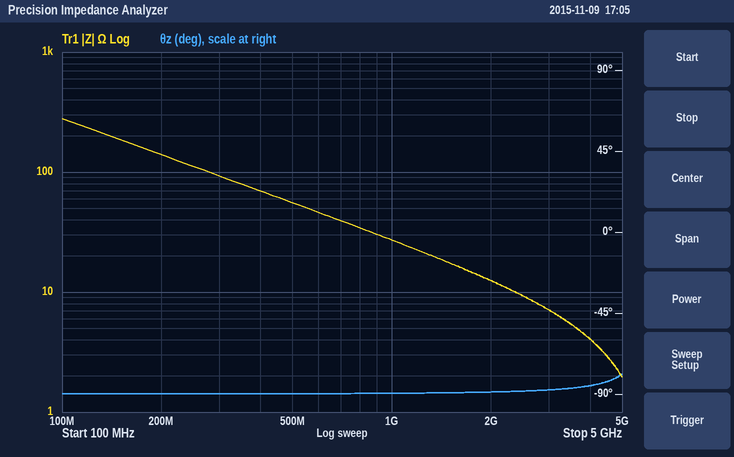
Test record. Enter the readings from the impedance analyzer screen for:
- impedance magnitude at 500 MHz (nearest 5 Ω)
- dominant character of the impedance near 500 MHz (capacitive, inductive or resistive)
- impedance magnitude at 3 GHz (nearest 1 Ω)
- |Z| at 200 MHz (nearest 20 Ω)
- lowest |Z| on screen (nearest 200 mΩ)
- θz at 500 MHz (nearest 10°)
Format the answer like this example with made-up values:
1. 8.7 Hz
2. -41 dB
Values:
1. 55 Ω
2. capacitive
3. 7 Ω
4. 140 Ω
5. 2.0 Ω
6. -90°
